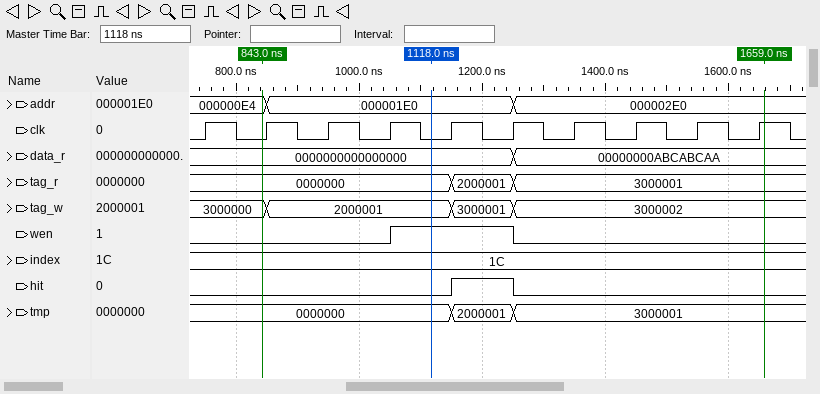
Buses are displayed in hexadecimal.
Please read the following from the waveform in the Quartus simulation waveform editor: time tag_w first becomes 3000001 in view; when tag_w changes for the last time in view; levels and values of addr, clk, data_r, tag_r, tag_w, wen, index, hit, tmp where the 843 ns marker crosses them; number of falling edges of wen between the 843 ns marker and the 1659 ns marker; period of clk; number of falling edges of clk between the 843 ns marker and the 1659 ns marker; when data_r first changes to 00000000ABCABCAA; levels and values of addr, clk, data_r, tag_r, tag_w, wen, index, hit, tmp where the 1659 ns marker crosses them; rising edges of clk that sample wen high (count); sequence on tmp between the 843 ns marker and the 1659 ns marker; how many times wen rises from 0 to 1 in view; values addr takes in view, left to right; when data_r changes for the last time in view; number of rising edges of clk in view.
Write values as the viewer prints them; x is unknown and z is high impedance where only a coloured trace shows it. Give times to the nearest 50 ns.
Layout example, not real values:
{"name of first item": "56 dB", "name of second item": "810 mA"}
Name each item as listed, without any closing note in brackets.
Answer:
{"time tag_w first becomes 3000001 in view": "1150 ns", "when tag_w changes for the last time in view": "1250 ns", "levels and values of addr, clk, data_r, tag_r, tag_w, wen, index, hit, tmp where the 843 ns marker crosses them": "addr=000000E4, clk=0, data_r=0000000000000000, tag_r=0000000, tag_w=3000000, wen=0, index=1C, hit=0, tmp=0000000", "number of falling edges of wen between the 843 ns marker and the 1659 ns marker": "1", "period of clk": "100 ns", "number of falling edges of clk between the 843 ns marker and the 1659 ns marker": "8", "when data_r first changes to 00000000ABCABCAA": "1250 ns", "levels and values of addr, clk, data_r, tag_r, tag_w, wen, index, hit, tmp where the 1659 ns marker crosses them": "addr=000002E0, clk=1, data_r=00000000ABCABCAA, tag_r=3000001, tag_w=3000002, wen=0, index=1C, hit=0, tmp=3000001", "rising edges of clk that sample wen high": "2", "sequence on tmp between the 843 ns marker and the 1659 ns marker": "0000000, 2000001, 3000001", "how many times wen rises from 0 to 1 in view": "1", "values addr takes in view, left to right": "000000E4, 000001E0, 000002E0", "when data_r changes for the last time in view": "1250 ns", "number of rising edges of clk in view": "10"}
